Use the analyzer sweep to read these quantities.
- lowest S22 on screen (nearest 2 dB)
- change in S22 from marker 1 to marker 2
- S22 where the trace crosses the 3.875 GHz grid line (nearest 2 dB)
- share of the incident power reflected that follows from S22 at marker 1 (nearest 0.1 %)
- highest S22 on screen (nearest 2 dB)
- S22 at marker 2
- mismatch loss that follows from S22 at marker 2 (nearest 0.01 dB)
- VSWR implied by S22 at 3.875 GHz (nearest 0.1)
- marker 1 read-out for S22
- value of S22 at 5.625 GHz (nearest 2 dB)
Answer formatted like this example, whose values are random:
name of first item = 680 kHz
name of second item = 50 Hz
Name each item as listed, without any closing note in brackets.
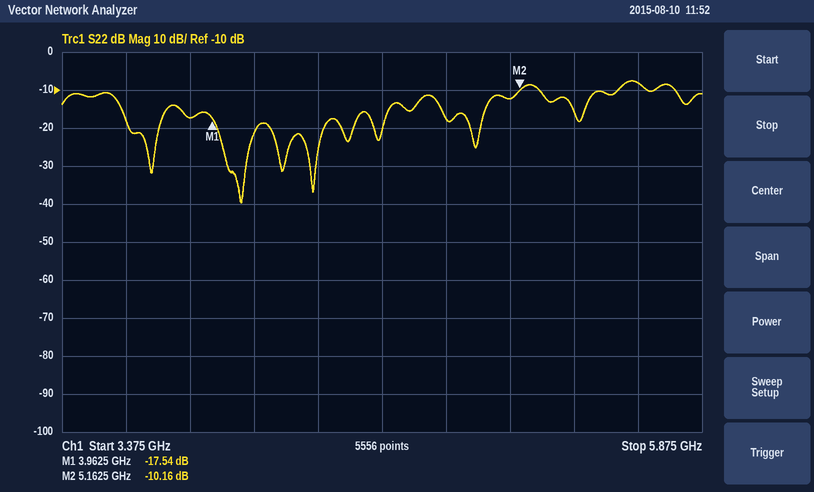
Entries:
lowest S22 on screen = -40 dB
change in S22 from marker 1 to marker 2 = 7.38 dB
S22 where the trace crosses the 3.875 GHz grid line = -18 dB
share of the incident power reflected that follows from S22 at marker 1 = 1.8 %
highest S22 on screen = -8 dB
S22 at marker 2 = -10.16 dB
mismatch loss that follows from S22 at marker 2 = 0.44 dB
VSWR implied by S22 at 3.875 GHz = 1.3
marker 1 read-out for S22 = -17.54 dB
value of S22 at 5.625 GHz = -8 dB
